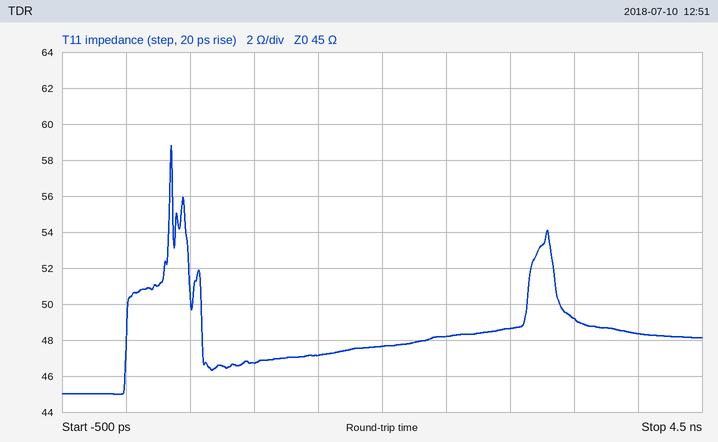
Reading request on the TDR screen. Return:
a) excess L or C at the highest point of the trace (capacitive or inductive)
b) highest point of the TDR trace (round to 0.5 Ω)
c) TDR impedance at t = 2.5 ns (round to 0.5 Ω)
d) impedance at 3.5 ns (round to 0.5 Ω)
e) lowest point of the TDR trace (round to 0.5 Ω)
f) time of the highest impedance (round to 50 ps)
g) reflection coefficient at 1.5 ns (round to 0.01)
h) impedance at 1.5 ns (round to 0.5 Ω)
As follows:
inductive
59.0 Ω
48.0 Ω
49.0 Ω
45.0 Ω
350 ps
+0.02
47.0 Ω
